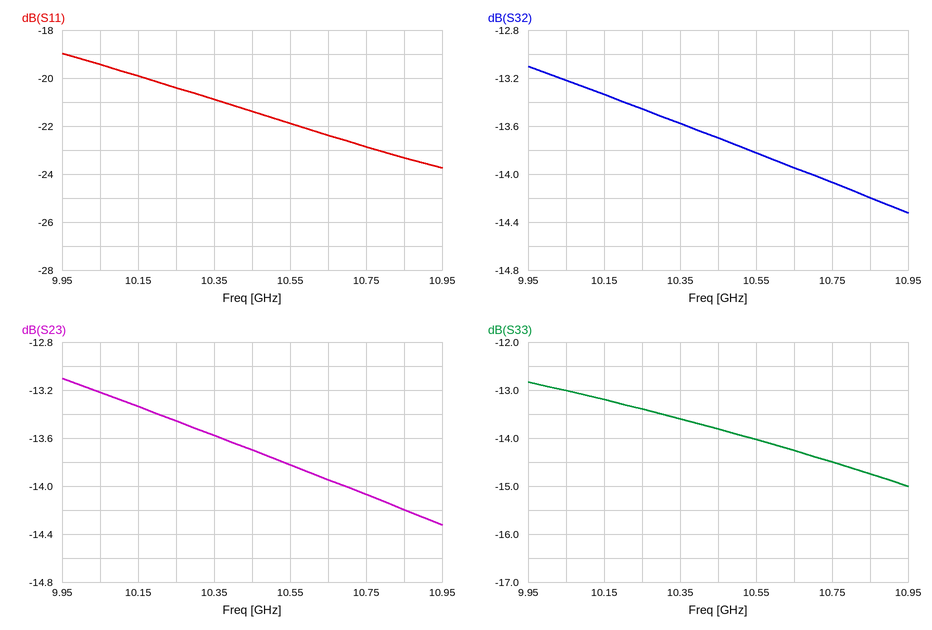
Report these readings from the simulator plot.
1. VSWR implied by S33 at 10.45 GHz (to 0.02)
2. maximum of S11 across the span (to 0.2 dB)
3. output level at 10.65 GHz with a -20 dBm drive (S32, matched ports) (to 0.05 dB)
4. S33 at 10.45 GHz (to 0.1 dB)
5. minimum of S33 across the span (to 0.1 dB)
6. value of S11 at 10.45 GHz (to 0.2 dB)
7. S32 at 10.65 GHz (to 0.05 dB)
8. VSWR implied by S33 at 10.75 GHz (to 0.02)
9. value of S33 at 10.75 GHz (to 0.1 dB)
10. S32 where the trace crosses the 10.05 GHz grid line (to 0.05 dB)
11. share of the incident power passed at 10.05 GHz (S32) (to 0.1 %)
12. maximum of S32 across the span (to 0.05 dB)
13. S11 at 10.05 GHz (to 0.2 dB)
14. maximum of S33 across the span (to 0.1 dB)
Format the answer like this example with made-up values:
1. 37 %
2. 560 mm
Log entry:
1. 1.52
2. -19.0 dB
3. -33.95 dBm
4. -13.8 dB
5. -15.0 dB
6. -21.4 dB
7. -13.95 dB
8. 1.46
9. -14.5 dB
10. -13.20 dB
11. 4.8 %
12. -13.10 dB
13. -19.4 dB
14. -12.8 dB
